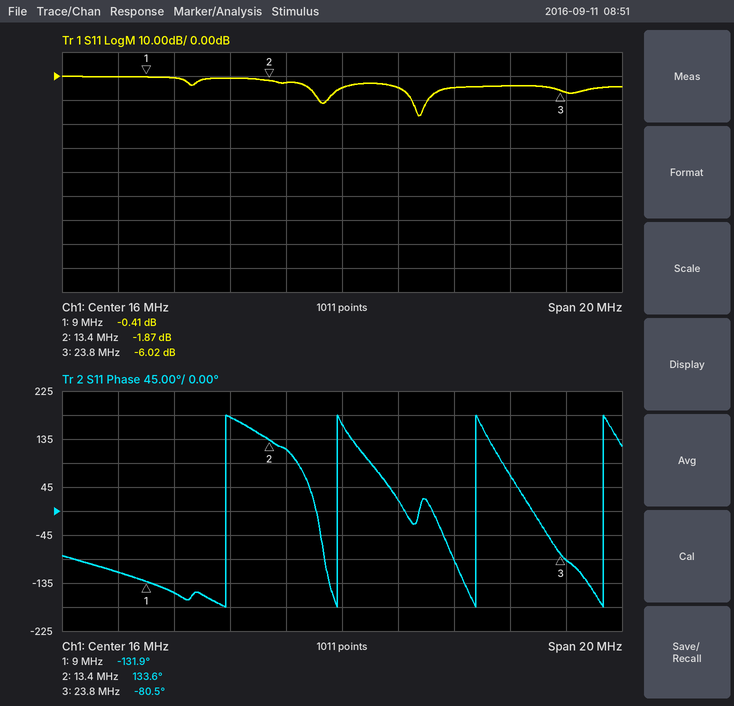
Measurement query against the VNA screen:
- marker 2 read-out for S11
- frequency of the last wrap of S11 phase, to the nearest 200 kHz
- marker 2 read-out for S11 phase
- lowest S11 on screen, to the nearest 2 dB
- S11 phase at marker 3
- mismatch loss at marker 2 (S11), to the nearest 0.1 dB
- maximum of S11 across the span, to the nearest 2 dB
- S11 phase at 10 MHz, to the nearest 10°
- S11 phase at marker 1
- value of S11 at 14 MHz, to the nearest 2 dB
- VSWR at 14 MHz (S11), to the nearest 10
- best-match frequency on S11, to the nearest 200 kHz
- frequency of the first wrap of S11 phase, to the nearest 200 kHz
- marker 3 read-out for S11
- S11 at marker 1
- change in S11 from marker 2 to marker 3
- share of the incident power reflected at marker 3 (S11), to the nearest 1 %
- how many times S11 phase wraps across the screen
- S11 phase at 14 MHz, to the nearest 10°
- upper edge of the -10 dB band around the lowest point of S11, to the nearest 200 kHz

-1.87 dB
25.4 MHz
133.6°
-16 dB
-80.5°
4.6 dB
0 dB
-150°
-131.9°
-2 dB
10
18.8 MHz
11.8 MHz
-6.02 dB
-0.41 dB
-4.15 dB
25 %
4
120°
19.0 MHz
